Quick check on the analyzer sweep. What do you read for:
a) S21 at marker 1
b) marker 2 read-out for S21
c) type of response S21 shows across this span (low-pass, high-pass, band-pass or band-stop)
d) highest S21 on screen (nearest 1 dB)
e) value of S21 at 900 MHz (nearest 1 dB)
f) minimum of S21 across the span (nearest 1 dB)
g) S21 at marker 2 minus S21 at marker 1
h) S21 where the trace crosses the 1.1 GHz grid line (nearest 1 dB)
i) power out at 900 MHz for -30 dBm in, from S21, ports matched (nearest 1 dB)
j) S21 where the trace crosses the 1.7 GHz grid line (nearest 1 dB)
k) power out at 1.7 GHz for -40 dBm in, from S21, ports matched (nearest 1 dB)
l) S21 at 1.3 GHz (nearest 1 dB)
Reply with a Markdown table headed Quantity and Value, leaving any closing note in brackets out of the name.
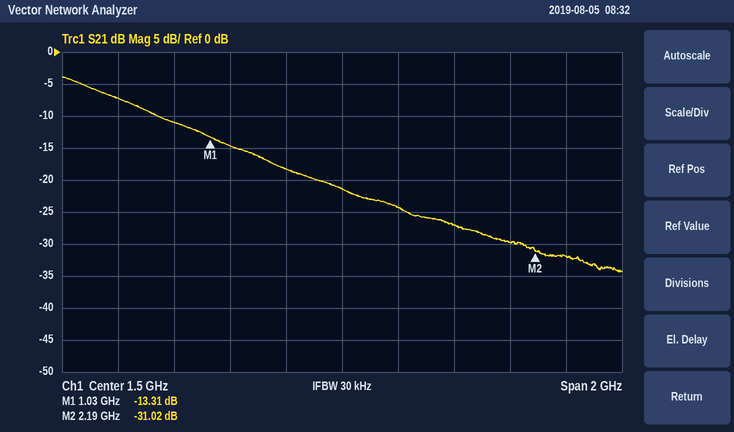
| Quantity | Value |
|---|---|
| S21 at marker 1 | -13.31 dB |
| marker 2 read-out for S21 | -31.02 dB |
| type of response S21 shows across this span | low-pass |
| highest S21 on screen | -4 dB |
| value of S21 at 900 MHz | -11 dB |
| minimum of S21 across the span | -34 dB |
| S21 at marker 2 minus S21 at marker 1 | -17.71 dB |
| S21 where the trace crosses the 1.1 GHz grid line | -15 dB |
| power out at 900 MHz for -30 dBm in, from S21, ports matched | -41 dBm |
| S21 where the trace crosses the 1.7 GHz grid line | -24 dB |
| power out at 1.7 GHz for -40 dBm in, from S21, ports matched | -64 dBm |
| S21 at 1.3 GHz | -18 dB |
